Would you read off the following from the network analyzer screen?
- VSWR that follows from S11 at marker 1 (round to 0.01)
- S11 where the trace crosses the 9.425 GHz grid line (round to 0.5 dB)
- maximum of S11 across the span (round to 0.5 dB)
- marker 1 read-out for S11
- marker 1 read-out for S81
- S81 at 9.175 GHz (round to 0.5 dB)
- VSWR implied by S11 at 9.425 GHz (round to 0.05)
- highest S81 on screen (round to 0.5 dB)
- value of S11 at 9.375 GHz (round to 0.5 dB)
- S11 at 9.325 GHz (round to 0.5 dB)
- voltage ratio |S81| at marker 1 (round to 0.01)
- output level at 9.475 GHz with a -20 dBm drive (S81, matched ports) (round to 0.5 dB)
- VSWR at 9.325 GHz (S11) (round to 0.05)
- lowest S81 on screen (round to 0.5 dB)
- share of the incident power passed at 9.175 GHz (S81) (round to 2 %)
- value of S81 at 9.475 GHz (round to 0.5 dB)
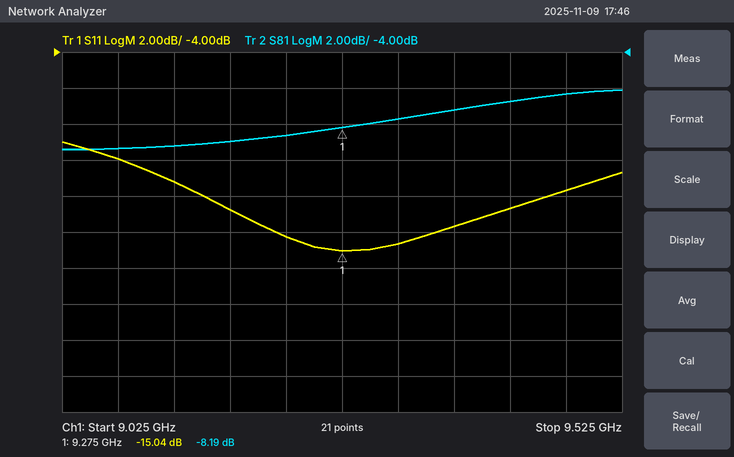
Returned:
1.43
-12.5 dB
-9.0 dB
-15.04 dB
-8.19 dB
-9.0 dB
1.60
-6.0 dB
-13.5 dB
-14.5 dB
0.39
-26.5 dBm
1.45
-9.5 dB
12 %
-6.5 dB
